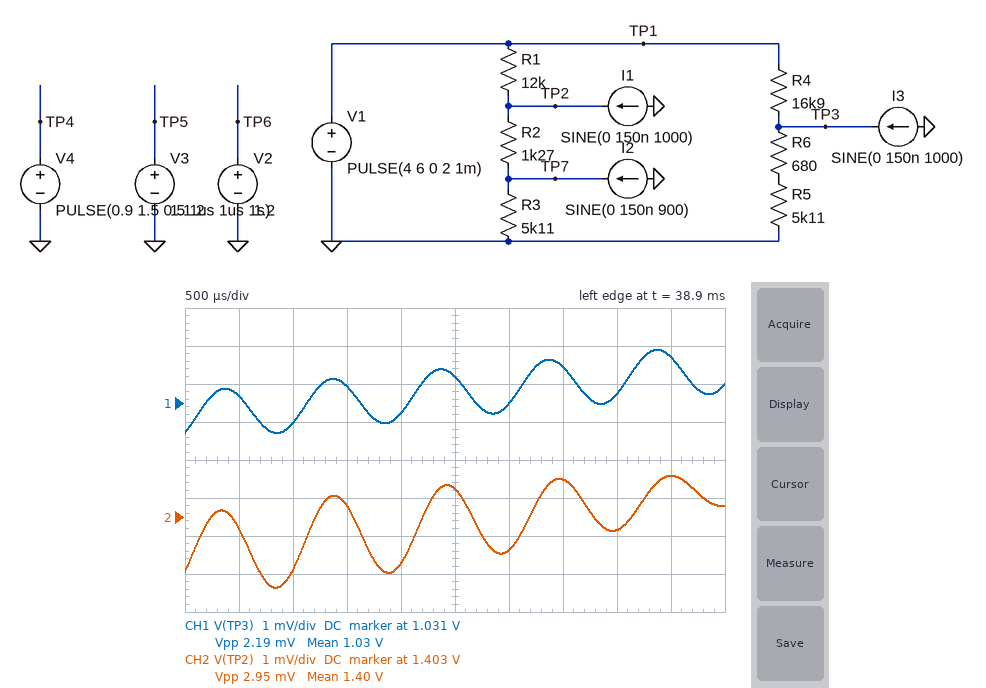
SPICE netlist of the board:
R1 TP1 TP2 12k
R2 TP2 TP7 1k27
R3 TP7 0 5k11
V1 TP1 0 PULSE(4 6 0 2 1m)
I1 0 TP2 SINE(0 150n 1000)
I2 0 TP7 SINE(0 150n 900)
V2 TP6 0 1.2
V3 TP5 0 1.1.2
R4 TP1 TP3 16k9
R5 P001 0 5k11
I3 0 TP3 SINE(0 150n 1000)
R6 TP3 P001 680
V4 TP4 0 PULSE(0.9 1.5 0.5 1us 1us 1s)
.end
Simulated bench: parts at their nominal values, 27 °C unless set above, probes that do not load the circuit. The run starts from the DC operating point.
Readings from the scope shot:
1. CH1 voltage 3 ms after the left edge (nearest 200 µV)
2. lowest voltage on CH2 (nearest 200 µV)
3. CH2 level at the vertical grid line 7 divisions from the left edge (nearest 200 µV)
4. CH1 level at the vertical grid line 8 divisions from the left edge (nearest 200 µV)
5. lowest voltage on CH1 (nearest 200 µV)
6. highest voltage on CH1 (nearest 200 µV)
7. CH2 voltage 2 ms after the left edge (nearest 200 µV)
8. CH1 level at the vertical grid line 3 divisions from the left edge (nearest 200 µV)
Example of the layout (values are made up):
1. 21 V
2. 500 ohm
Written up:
1. 1.0310 V
2. 1.4012 V
3. 1.4040 V
4. 1.0312 V
5. 1.0302 V
6. 1.0324 V
7. 1.4018 V
8. 1.0314 V
